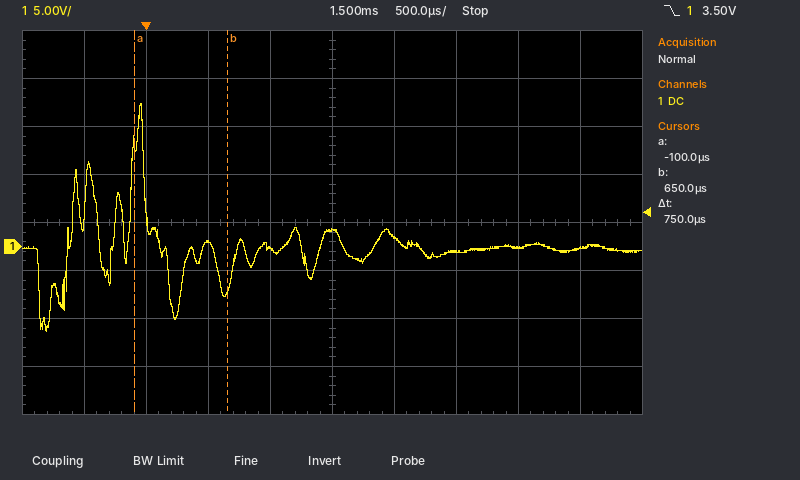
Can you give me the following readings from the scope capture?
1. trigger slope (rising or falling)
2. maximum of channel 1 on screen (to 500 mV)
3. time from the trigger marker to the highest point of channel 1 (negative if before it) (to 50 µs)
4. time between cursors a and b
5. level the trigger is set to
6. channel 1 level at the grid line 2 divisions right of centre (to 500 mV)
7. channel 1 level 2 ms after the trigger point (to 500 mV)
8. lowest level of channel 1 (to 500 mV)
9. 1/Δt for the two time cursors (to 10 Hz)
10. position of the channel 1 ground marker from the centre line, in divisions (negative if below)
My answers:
falling
15.0 V
-50 µs
750 µs
3.50 V
-500 mV
1.0 V
-9.0 V
1.33 kHz
-0.5 div
